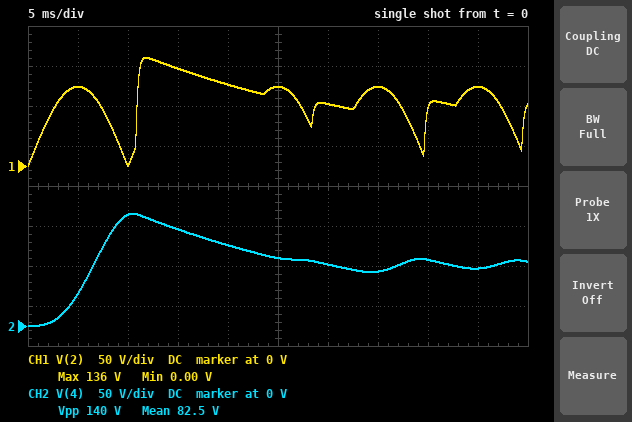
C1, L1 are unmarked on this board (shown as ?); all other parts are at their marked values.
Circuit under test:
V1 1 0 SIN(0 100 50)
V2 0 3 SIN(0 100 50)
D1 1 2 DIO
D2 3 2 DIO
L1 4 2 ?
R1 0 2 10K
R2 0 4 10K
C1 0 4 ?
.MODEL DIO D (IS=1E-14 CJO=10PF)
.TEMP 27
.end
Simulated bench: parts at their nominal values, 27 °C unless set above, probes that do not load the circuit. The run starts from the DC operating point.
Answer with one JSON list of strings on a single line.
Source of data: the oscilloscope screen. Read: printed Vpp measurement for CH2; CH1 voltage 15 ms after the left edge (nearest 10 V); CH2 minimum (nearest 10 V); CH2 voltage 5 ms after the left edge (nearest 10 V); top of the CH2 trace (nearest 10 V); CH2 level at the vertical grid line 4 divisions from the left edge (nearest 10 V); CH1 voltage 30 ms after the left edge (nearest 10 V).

["140 V", "120 V", "0 V", "40 V", "140 V", "100 V", "80 V"]
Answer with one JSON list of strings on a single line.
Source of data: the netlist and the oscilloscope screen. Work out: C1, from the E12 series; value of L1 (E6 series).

["5.6 µF", "2.2 H"]
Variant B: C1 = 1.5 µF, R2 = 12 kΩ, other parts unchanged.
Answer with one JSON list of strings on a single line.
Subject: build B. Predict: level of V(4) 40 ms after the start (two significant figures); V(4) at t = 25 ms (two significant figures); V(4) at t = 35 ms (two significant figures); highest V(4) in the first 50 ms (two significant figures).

["90 V", "68 V", "68 V", "160 V"]
